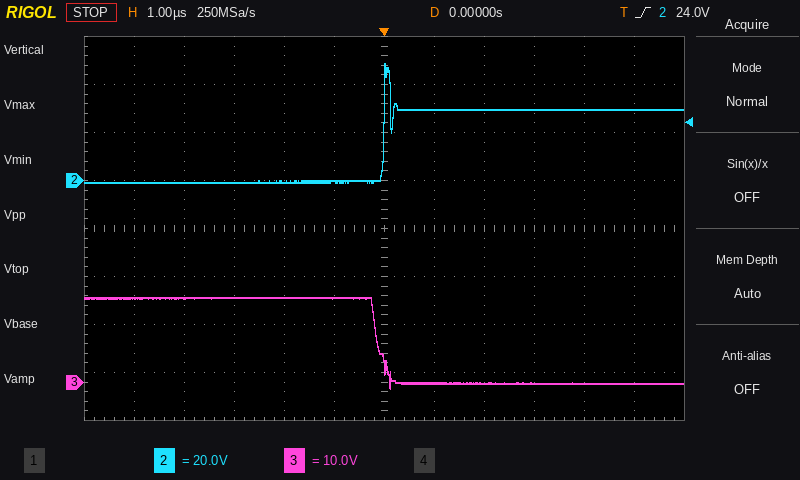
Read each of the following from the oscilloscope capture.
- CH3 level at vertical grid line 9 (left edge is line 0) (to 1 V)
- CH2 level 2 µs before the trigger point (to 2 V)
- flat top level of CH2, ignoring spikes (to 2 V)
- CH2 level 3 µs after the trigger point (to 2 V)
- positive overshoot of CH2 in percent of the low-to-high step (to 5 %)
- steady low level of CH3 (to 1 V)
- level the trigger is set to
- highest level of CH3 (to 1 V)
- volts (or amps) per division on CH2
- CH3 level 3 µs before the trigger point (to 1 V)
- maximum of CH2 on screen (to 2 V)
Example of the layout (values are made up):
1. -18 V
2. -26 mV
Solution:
1. 0 V
2. 0 V
3. 30 V
4. 30 V
5. 65 %
6. 0 V
7. 24.0 V
8. 18 V
9. 20 V
10. 18 V
11. 48 V
